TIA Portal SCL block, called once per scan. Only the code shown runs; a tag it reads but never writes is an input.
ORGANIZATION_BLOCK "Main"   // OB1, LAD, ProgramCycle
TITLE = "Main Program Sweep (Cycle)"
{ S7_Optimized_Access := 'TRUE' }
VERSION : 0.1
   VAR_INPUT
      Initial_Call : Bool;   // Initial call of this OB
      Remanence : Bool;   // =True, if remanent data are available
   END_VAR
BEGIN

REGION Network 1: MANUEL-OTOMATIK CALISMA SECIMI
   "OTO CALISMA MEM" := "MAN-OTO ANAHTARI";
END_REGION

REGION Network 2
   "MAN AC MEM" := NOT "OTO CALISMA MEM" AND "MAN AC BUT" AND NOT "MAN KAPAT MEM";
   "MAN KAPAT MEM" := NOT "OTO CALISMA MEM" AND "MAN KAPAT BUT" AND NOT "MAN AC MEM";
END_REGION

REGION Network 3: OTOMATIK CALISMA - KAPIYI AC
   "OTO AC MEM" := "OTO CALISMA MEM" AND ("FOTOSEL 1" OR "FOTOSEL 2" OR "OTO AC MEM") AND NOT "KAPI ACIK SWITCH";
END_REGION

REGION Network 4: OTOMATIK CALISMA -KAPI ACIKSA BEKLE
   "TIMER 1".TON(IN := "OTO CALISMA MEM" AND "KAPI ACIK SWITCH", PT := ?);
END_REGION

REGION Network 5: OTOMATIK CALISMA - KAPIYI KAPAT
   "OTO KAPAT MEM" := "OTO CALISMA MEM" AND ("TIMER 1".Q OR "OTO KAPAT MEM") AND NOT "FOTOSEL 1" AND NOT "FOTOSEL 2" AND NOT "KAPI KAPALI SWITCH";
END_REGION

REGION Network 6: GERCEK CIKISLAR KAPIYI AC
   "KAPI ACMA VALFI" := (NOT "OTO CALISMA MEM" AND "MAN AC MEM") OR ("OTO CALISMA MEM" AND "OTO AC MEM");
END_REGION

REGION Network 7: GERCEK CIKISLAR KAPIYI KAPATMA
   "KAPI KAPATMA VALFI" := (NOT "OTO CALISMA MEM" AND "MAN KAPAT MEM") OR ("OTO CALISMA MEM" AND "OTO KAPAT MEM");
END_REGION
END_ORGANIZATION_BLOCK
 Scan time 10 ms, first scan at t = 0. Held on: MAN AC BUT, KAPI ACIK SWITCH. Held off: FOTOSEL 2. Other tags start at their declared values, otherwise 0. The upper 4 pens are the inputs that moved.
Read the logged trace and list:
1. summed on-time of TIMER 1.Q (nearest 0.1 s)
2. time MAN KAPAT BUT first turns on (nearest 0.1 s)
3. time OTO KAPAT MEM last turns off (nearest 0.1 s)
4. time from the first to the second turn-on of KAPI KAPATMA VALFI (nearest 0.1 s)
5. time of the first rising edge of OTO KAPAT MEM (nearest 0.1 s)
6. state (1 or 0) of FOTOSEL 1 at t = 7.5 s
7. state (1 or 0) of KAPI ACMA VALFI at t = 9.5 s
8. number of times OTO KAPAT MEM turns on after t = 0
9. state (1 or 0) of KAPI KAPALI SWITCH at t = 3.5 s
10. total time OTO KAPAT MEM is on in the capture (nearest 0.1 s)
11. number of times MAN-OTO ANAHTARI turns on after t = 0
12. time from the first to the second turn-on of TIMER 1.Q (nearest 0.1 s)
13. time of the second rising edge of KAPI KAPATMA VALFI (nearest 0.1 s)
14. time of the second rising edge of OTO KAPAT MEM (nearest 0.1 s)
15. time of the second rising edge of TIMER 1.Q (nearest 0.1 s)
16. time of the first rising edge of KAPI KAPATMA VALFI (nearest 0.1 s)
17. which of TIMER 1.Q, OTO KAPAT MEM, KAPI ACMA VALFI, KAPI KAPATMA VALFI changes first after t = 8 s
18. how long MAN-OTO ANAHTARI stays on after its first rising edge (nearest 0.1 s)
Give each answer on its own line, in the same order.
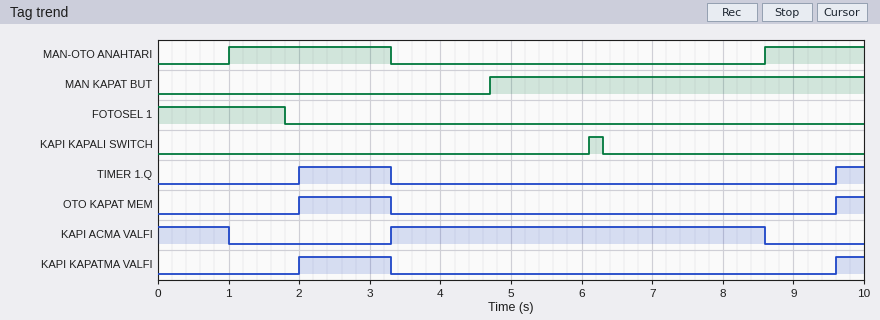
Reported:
1.7 s
4.7 s
3.3 s
7.6 s
2.0 s
0
0
2
0
1.7 s
2
7.6 s
9.6 s
9.6 s
9.6 s
2.0 s
KAPI ACMA VALFI
2.3 s
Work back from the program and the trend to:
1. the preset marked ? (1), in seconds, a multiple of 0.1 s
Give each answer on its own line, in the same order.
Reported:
1.0 s
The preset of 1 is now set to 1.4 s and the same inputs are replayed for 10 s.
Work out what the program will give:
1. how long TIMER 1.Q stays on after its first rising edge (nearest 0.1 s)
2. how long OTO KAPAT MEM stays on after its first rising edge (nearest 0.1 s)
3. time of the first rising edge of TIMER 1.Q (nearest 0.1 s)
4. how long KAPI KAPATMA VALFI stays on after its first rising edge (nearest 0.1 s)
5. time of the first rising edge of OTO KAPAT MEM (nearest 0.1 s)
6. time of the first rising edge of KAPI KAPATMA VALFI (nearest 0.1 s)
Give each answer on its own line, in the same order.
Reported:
0.9 s
0.9 s
2.4 s
0.9 s
2.4 s
2.4 s
